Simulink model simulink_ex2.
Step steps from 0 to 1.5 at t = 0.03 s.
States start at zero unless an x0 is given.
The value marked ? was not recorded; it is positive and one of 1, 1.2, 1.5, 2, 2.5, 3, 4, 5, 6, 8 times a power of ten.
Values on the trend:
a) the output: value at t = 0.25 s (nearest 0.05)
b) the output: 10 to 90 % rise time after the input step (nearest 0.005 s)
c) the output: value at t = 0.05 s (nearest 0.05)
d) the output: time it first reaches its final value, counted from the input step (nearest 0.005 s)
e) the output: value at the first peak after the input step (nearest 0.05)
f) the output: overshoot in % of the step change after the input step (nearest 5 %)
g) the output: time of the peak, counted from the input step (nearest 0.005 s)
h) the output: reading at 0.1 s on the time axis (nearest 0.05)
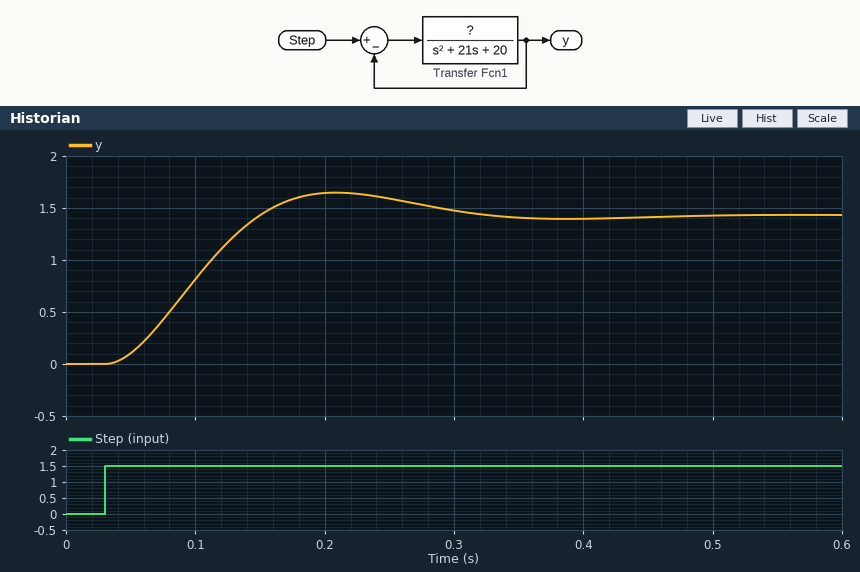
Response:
1.60
0.080 s
0.10
0.120 s
1.65
15 %
0.180 s
0.80
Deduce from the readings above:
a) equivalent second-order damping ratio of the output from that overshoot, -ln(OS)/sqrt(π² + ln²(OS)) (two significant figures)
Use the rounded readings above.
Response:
0.52
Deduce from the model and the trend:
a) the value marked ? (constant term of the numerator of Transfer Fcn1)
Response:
400
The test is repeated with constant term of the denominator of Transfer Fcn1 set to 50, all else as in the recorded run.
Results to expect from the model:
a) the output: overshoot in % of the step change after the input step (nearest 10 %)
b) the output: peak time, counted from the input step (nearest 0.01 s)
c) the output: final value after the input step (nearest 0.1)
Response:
20 %
0.17 s
1.3
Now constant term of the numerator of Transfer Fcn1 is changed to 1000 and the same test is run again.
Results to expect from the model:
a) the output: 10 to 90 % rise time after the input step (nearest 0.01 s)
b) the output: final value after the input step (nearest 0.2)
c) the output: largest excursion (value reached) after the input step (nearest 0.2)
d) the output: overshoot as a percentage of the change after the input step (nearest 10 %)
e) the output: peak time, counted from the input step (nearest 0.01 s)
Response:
0.04 s
1.4
2.0
30 %
0.10 s
